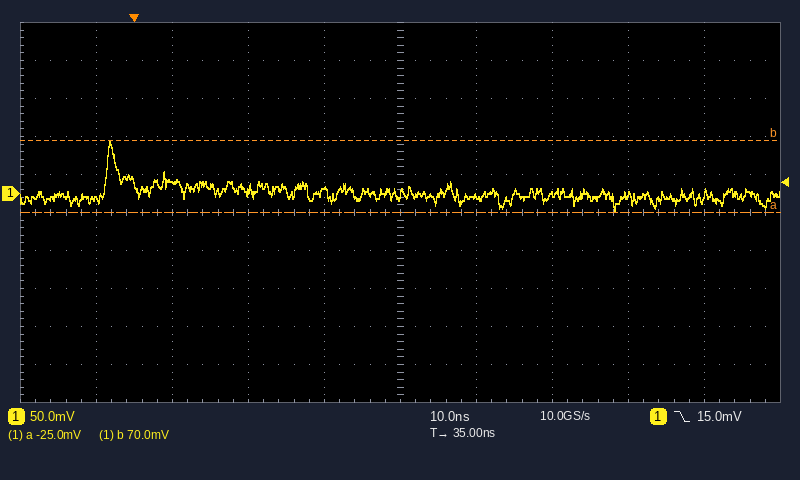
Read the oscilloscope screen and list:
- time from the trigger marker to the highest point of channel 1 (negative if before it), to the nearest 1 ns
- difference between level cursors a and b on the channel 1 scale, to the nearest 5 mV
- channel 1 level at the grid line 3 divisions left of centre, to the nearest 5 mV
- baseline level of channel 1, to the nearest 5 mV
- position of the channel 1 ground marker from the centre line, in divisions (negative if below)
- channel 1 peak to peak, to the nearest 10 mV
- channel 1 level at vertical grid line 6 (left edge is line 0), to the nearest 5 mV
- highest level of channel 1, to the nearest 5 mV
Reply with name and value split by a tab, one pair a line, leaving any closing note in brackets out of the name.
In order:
time from the trigger marker to the highest point of channel 1 (negative if before it), to the nearest 1 ns	-3 ns
difference between level cursors a and b on the channel 1 scale, to the nearest 5 mV	95 mV
channel 1 level at the grid line 3 divisions left of centre, to the nearest 5 mV	15 mV
baseline level of channel 1, to the nearest 5 mV	0 mV
position of the channel 1 ground marker from the centre line, in divisions	+0.5 div
channel 1 peak to peak, to the nearest 10 mV	90 mV
channel 1 level at vertical grid line 6 (left edge is line 0), to the nearest 5 mV	-5 mV
highest level of channel 1, to the nearest 5 mV	70 mV
